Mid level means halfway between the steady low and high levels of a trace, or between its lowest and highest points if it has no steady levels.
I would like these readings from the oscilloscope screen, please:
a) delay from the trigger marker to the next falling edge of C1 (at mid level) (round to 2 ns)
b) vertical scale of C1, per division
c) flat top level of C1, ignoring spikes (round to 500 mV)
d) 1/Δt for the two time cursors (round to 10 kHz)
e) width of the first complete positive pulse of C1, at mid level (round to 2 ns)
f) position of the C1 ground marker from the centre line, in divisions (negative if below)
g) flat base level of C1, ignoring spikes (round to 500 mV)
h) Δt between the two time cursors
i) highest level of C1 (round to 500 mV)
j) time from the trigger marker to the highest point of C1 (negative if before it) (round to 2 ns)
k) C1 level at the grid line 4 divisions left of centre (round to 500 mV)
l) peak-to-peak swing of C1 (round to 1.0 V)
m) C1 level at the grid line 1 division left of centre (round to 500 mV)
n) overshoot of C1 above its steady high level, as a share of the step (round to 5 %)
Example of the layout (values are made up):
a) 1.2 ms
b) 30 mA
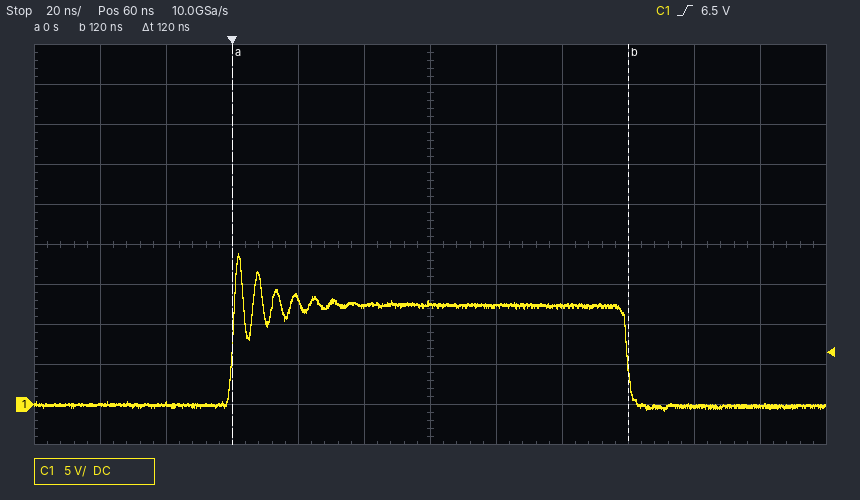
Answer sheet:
a) 120 ns
b) 5 V
c) 12.5 V
d) 8.33 MHz
e) 120 ns
f) -4.0 div
g) 0.0 V
h) 120 ns
i) 19.0 V
j) +2 ns
k) 0.0 V
l) 20.0 V
m) 12.5 V
n) 50 %
